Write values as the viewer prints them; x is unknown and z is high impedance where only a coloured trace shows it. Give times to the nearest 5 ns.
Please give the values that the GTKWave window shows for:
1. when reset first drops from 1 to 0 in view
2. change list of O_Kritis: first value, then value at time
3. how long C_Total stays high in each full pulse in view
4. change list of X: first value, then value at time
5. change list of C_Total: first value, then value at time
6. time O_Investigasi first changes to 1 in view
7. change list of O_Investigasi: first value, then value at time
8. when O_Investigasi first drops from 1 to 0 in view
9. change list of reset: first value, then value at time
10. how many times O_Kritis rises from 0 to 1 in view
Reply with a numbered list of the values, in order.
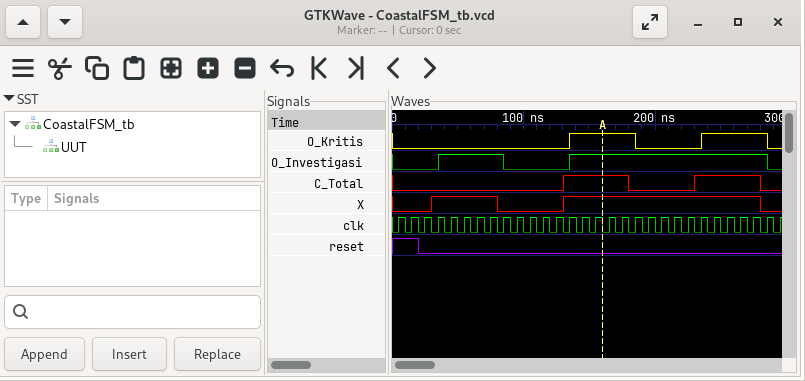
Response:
1. 20 ns
2. 0, 1 at 135 ns, 0 at 185 ns, 1 at 235 ns, 0 at 285 ns
3. 50 ns, 50 ns
4. 0, 1 at 30 ns, 0 at 80 ns, 1 at 130 ns, 0 at 280 ns
5. 0, 1 at 130 ns, 0 at 180 ns, 1 at 230 ns, 0 at 280 ns
6. 35 ns
7. 0, 1 at 35 ns, 0 at 85 ns, 1 at 135 ns, 0 at 285 ns
8. 85 ns
9. 1, 0 at 20 ns
10. 2
